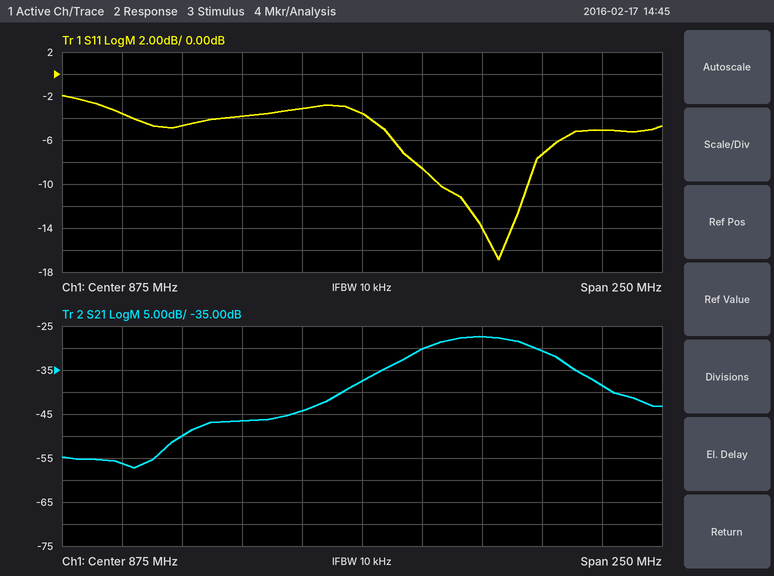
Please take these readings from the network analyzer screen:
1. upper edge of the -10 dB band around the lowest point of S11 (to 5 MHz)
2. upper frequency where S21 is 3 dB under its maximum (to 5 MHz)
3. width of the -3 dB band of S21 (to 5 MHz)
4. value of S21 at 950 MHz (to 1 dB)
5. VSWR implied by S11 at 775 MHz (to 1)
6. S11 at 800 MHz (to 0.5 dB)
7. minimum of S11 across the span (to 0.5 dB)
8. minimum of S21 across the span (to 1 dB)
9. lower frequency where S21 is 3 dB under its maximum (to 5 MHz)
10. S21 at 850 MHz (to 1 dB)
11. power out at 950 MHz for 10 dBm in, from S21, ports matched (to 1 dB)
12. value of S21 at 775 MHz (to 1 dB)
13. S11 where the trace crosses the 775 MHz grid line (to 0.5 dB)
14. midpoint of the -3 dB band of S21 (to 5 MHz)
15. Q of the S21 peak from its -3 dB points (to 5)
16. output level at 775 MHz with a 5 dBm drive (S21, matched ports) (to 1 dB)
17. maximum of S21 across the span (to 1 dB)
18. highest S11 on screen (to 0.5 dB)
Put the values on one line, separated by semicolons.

945 MHz; 950 MHz; 50 MHz; -31 dB; 5; -4.5 dB; -17.0 dB; -57 dB; 900 MHz; -44 dB; -21 dBm; -56 dB; -3.5 dB; 925 MHz; 20; -51 dBm; -27 dB; -2.0 dB
